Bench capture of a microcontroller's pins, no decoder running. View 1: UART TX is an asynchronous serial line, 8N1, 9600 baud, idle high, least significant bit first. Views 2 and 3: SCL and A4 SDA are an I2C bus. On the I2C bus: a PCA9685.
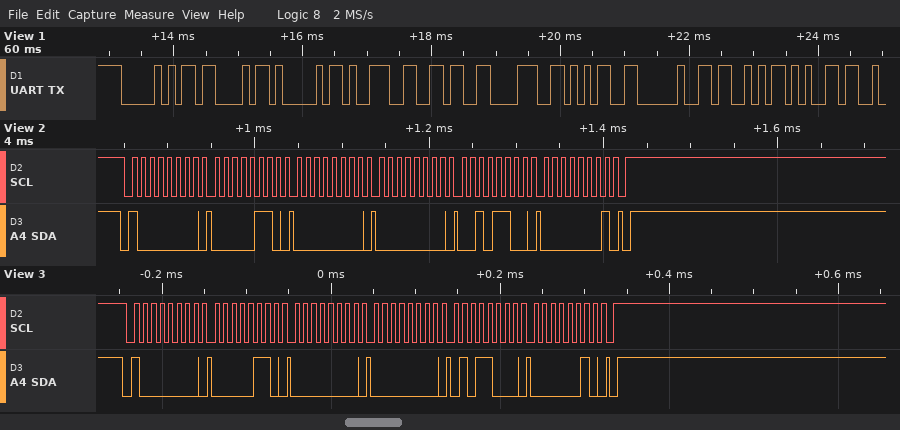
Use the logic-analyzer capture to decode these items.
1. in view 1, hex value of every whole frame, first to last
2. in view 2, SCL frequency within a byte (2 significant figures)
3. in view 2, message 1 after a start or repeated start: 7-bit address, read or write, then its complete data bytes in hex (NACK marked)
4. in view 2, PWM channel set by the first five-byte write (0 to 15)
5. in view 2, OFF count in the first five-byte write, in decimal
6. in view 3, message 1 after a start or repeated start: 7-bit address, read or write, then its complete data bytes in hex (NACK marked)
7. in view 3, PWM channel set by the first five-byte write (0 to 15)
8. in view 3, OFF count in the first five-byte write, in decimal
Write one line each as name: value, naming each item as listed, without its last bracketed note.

in view 1, hex value of every whole frame, first to last: 50 43 41 39 36 38 35 20 53 65
in view 2, SCL frequency within a byte: 100 kHz
in view 2, message 1 after a start or repeated start: 7-bit address, read or write, then its complete data bytes in hex: 0x40 write: 06 00 00 2C 01
in view 2, PWM channel set by the first five-byte write: 0
in view 2, OFF count in the first five-byte write, in decimal: 300
in view 3, message 1 after a start or repeated start: 7-bit address, read or write, then its complete data bytes in hex: 0x40 write: 06 00 00 58 02
in view 3, PWM channel set by the first five-byte write: 0
in view 3, OFF count in the first five-byte write, in decimal: 600
